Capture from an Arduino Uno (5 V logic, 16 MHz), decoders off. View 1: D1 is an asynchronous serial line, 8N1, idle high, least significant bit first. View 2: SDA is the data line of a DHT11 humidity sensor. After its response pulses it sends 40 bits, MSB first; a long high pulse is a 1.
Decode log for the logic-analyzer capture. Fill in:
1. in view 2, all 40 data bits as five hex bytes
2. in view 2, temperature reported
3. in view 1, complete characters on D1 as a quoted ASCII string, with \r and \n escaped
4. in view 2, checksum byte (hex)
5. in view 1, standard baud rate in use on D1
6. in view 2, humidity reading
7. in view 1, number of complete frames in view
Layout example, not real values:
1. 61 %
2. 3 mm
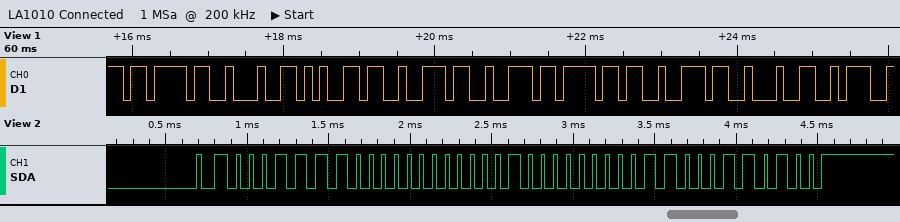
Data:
1. 1E 00 10 06 34
2. 16.6 °C
3. "{\"error\":"
4. 0x34
5. 9600 baud
6. 30 %
7. 9
